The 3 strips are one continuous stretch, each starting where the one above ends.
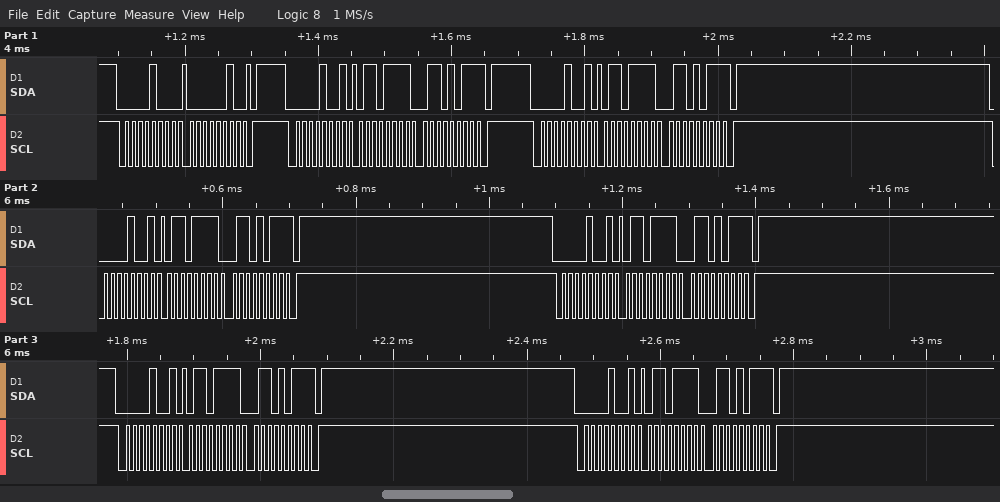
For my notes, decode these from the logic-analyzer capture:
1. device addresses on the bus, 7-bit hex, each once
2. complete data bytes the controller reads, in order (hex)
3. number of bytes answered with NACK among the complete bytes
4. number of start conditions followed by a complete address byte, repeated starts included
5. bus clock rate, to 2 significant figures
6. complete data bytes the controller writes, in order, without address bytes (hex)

0x04
6F 6B 6F 6B 6F 6B 6F 6B 6F 6B 6F 6B
6
7
100 kHz
02
